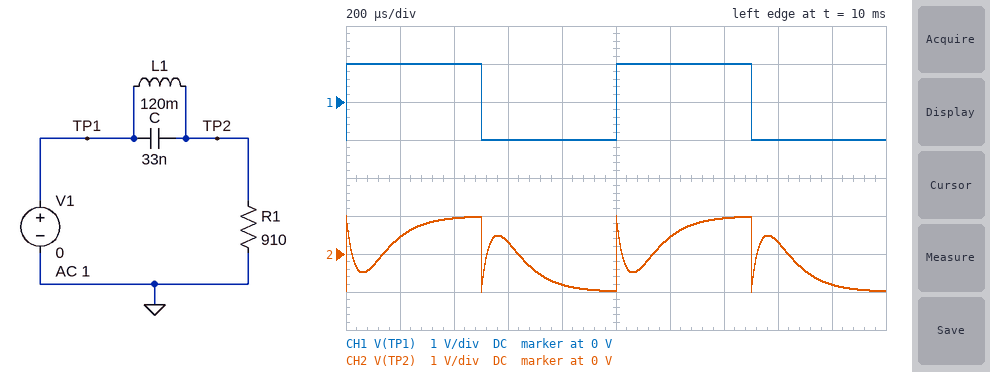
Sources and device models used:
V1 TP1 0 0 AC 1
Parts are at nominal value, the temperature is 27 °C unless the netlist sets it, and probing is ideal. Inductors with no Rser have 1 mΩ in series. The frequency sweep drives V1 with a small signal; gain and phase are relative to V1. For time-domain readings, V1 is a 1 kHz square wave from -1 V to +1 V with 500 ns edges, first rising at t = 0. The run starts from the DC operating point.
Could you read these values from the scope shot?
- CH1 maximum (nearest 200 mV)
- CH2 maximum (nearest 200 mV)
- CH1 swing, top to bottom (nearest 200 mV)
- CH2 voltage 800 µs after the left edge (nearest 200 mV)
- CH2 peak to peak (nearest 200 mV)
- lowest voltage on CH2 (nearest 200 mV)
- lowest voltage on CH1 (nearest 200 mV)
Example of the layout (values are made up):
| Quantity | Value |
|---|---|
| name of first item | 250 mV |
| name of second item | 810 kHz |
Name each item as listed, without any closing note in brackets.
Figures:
| Quantity | Value |
|---|---|
| CH1 maximum | 1.0 V |
| CH2 maximum | 1.0 V |
| CH1 swing, top to bottom | 2.0 V |
| CH2 voltage 800 µs after the left edge | -800 mV |
| CH2 peak to peak | 2.0 V |
| lowest voltage on CH2 | -1.0 V |
| lowest voltage on CH1 | -1.0 V |
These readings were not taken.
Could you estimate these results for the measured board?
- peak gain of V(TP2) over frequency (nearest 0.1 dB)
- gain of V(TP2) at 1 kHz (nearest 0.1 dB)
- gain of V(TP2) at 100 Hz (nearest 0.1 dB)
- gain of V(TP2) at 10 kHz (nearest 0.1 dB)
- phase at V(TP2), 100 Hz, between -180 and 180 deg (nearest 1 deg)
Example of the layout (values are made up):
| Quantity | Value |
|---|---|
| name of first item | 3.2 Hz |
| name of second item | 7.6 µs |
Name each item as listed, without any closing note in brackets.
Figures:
| Quantity | Value |
|---|---|
| peak gain of V(TP2) over frequency | 0 dB |
| gain of V(TP2) at 1 kHz | -2.9 dB |
| gain of V(TP2) at 100 Hz | 0 dB |
| gain of V(TP2) at 10 kHz | -1.2 dB |
| phase at V(TP2), 100 Hz, between -180 and 180 deg | -5 deg |
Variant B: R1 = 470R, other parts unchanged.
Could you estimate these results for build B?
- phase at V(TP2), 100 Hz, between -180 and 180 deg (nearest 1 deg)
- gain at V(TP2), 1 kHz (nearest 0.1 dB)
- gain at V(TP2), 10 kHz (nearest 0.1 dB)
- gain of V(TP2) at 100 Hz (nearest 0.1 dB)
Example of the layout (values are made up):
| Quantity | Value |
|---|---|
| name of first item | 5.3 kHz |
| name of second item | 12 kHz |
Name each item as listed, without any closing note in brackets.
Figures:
| Quantity | Value |
|---|---|
| phase at V(TP2), 100 Hz, between -180 and 180 deg | -9 deg |
| gain at V(TP2), 1 kHz | -6.6 dB |
| gain at V(TP2), 10 kHz | -3.4 dB |
| gain of V(TP2) at 100 Hz | -0.1 dB |
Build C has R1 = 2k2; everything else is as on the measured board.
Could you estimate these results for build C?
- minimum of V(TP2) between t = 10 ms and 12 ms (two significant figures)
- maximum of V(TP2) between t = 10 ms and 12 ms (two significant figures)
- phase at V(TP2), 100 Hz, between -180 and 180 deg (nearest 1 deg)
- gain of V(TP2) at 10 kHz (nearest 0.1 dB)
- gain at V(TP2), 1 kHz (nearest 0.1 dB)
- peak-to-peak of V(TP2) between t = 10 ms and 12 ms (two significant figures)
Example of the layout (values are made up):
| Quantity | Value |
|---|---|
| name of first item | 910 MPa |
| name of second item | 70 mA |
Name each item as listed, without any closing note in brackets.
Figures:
| Quantity | Value |
|---|---|
| minimum of V(TP2) between t = 10 ms and 12 ms | -1.2 V |
| maximum of V(TP2) between t = 10 ms and 12 ms | 1.2 V |
| phase at V(TP2), 100 Hz, between -180 and 180 deg | -2 deg |
| gain of V(TP2) at 10 kHz | -0.2 dB |
| gain at V(TP2), 1 kHz | -0.7 dB |
| peak-to-peak of V(TP2) between t = 10 ms and 12 ms | 2.4 V |
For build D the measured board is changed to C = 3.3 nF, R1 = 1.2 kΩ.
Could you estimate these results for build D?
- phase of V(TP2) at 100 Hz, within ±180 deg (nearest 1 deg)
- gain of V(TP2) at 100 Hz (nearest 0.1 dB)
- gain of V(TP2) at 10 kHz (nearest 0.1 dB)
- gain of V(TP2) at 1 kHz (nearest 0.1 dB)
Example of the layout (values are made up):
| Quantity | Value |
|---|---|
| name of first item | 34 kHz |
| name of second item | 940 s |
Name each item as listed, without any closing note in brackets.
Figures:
| Quantity | Value |
|---|---|
| phase of V(TP2) at 100 Hz, within ±180 deg | -4 deg |
| gain of V(TP2) at 100 Hz | 0 dB |
| gain of V(TP2) at 10 kHz | -21.0 dB |
| gain of V(TP2) at 1 kHz | -1.5 dB |
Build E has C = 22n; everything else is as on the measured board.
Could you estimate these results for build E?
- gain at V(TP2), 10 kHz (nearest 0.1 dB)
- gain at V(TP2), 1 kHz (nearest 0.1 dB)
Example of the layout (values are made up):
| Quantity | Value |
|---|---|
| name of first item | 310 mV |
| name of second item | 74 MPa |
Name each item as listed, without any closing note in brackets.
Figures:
| Quantity | Value |
|---|---|
| gain at V(TP2), 10 kHz | -2.5 dB |
| gain at V(TP2), 1 kHz | -2.7 dB |
